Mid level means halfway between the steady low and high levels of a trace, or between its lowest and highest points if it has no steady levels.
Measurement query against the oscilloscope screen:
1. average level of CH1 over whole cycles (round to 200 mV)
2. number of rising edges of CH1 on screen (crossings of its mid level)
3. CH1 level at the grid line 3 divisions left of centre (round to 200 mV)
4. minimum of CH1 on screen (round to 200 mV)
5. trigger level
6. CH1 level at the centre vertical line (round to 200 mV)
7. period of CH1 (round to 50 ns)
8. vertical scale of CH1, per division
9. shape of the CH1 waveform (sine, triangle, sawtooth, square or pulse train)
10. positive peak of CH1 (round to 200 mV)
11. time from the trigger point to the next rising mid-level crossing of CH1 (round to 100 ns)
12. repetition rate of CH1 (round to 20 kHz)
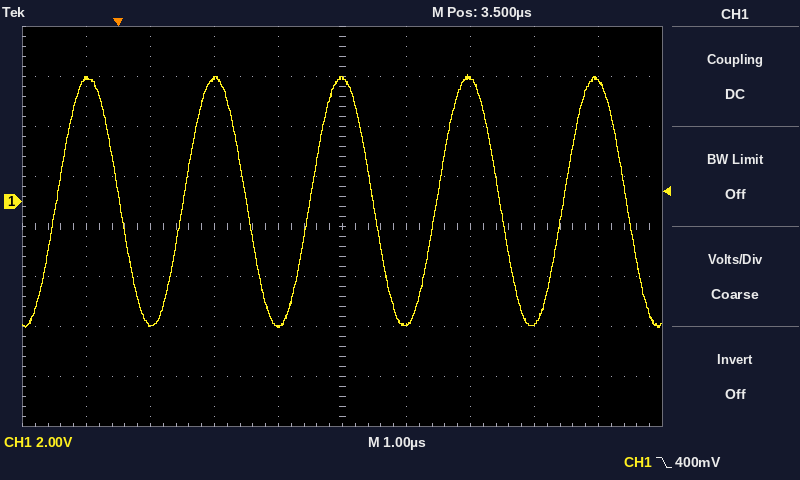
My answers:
0.0 V
5
-5.0 V
-5.0 V
400 mV
5.0 V
2.00 µs
2 V
sine
5.0 V
1.0 µs
500 kHz
